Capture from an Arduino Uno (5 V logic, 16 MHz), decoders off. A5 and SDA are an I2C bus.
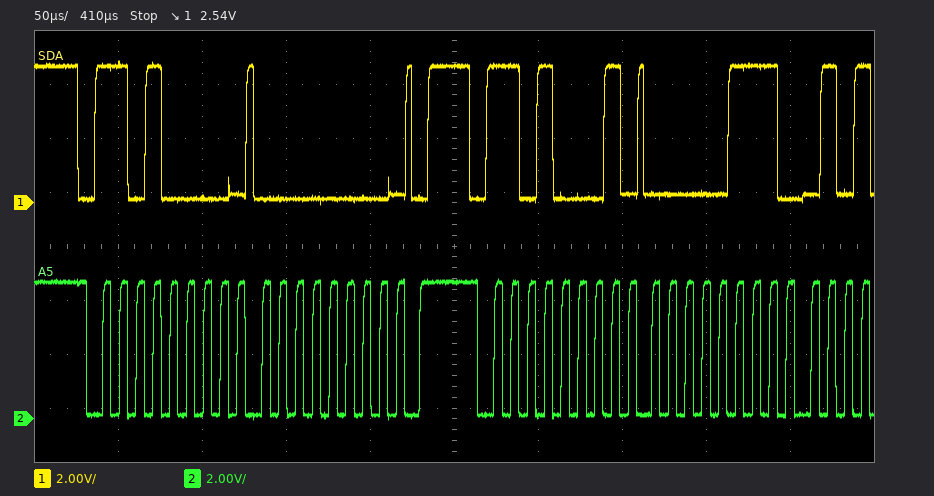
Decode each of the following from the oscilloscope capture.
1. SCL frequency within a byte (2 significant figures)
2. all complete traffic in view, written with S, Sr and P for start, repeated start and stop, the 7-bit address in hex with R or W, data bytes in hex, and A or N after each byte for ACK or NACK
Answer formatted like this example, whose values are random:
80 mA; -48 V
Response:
100 kHz; S 68W A 00 A P S 68R A 07 A
